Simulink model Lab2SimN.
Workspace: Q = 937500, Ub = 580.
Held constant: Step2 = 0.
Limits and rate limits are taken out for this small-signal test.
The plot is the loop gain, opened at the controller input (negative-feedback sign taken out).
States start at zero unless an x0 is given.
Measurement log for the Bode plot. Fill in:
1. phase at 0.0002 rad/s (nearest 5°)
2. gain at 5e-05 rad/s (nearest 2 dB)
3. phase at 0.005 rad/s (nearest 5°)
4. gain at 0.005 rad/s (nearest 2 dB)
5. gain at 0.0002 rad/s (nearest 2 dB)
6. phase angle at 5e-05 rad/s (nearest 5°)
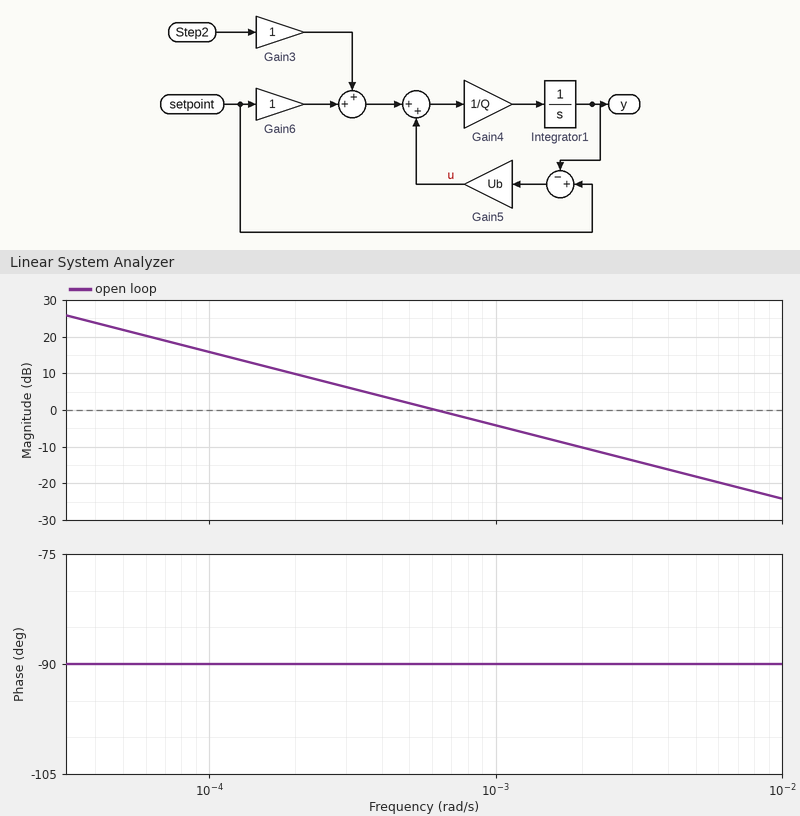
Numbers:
-90°
22 dB
-90°
-18 dB
10 dB
-90°
